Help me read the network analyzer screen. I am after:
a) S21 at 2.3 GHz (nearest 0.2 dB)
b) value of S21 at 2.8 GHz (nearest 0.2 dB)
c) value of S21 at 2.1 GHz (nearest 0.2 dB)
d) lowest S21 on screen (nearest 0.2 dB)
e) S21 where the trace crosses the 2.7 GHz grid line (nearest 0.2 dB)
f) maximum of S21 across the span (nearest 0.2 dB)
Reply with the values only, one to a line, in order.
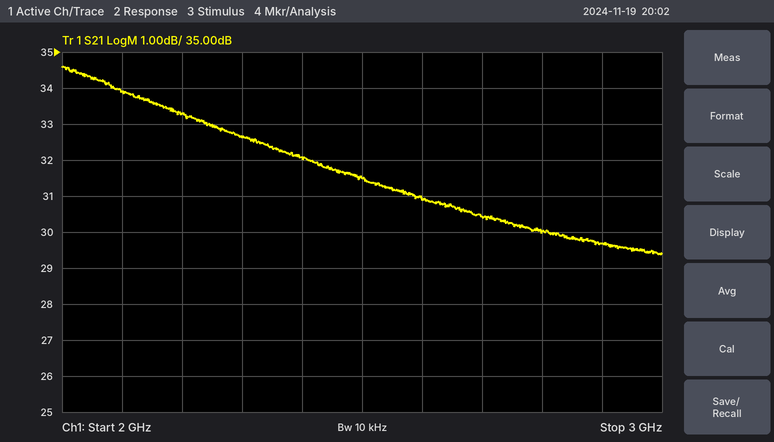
32.6 dB
30.0 dB
34.0 dB
29.4 dB
30.4 dB
34.6 dB
